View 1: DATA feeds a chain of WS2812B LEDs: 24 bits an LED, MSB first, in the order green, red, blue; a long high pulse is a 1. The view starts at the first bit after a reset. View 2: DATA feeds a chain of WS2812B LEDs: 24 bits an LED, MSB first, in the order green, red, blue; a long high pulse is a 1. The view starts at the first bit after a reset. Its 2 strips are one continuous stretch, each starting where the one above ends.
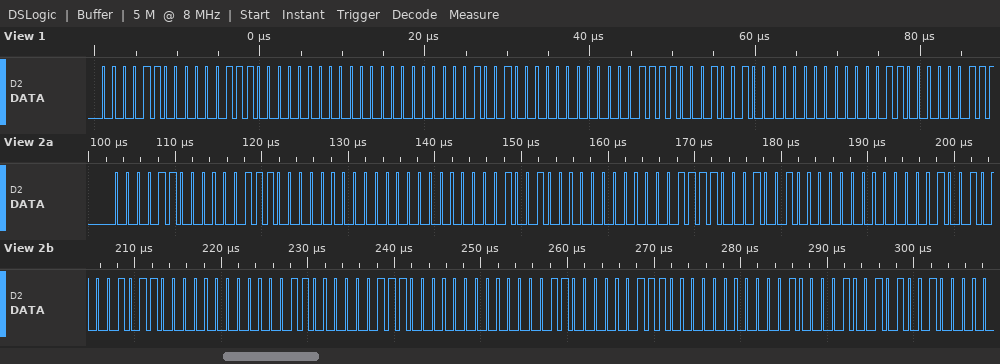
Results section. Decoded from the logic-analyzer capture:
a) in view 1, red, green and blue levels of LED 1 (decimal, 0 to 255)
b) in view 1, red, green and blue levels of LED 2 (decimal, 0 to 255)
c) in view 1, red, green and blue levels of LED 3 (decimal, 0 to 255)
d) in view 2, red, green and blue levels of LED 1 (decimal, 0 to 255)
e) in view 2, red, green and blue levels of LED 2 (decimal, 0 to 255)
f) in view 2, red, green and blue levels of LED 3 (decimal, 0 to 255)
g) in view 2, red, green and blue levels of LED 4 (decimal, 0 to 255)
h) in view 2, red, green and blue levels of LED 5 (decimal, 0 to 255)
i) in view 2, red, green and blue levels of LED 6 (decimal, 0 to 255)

14, 12, 0
9, 0, 0
18, 15, 0
14, 12, 0
9, 0, 0
18, 15, 0
11, 9, 0
14, 12, 0
14, 12, 0
